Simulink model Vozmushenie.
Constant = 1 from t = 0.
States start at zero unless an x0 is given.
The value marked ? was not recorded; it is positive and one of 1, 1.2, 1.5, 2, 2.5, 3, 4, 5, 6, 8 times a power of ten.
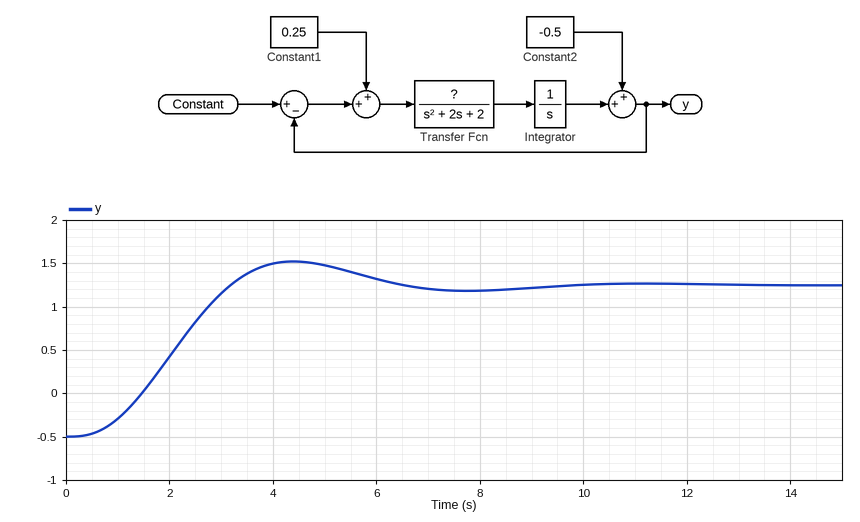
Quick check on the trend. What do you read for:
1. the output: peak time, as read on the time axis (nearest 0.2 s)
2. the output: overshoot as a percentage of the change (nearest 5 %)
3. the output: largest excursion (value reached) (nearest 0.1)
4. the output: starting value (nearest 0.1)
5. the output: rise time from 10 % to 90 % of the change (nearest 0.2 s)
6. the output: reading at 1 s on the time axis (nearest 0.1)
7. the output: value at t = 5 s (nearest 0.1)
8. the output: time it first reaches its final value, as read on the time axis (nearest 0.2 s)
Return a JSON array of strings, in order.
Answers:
["4.4 s", "15 %", "1.5", "-0.5", "2.0 s", "-0.3", "1.5", "3.2 s"]
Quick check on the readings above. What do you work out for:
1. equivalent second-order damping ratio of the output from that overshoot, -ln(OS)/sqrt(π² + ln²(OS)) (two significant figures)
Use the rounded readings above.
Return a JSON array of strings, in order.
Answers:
["0.52"]
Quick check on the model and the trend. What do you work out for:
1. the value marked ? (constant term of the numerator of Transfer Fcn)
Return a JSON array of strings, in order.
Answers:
["1.2"]
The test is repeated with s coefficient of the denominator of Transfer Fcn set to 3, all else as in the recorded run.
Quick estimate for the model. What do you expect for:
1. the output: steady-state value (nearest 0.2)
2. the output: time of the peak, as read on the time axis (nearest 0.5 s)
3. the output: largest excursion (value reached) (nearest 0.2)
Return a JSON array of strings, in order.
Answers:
["1.2", "5.5 s", "1.6"]
